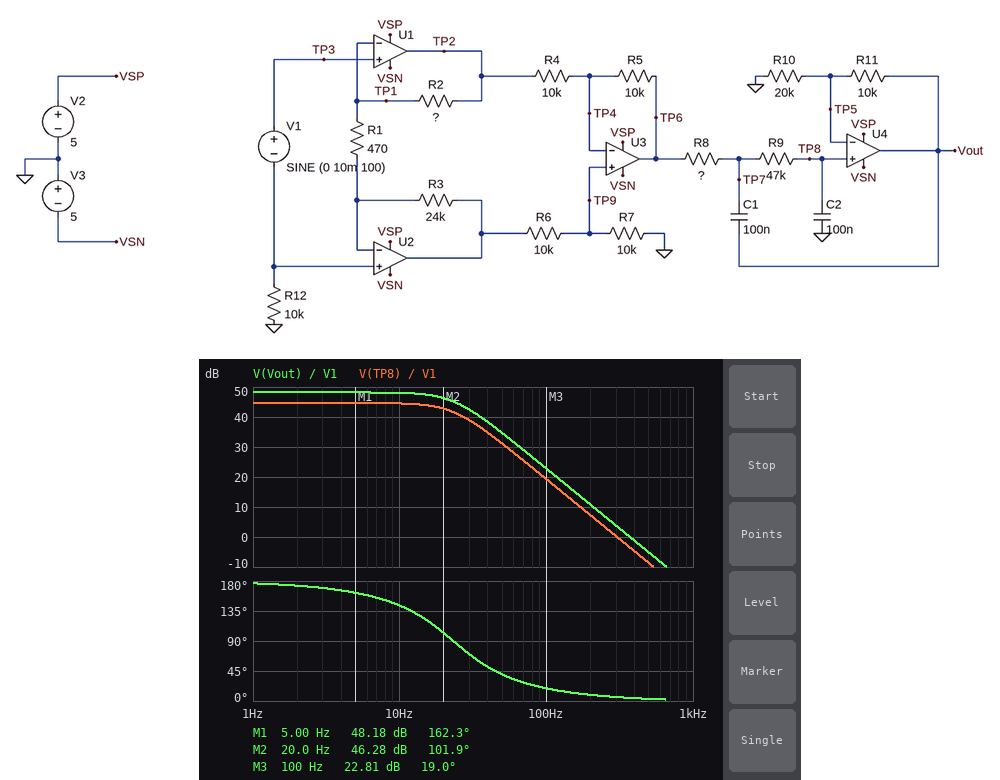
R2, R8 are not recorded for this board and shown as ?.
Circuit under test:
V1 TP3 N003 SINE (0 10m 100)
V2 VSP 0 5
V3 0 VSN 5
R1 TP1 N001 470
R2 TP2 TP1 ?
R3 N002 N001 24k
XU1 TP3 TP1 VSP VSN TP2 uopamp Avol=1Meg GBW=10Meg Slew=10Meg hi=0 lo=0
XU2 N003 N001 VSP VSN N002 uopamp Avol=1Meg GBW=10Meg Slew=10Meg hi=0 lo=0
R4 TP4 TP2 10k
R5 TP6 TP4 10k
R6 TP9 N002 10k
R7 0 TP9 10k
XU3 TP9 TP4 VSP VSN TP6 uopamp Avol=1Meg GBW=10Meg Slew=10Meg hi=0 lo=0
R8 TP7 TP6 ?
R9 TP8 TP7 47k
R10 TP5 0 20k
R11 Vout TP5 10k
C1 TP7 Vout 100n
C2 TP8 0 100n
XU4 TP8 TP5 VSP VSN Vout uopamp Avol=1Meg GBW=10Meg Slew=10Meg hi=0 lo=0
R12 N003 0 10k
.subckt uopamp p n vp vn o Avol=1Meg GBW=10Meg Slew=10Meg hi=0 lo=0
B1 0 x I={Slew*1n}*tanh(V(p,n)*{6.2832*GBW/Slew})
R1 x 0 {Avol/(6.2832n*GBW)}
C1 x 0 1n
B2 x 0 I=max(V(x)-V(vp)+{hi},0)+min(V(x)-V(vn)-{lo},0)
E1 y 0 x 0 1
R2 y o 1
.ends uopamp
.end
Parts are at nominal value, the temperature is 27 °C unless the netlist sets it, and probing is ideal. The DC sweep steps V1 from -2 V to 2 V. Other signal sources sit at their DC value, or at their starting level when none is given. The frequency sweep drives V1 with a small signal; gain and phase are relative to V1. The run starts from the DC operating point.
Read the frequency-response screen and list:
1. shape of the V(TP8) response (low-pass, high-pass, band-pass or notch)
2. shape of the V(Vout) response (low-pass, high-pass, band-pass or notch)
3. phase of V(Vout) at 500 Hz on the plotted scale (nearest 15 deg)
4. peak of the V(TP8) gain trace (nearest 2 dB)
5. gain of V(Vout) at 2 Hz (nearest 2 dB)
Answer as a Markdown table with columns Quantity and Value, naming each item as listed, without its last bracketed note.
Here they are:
| Quantity | Value |
|---|---|
| shape of the V(TP8) response | low-pass |
| shape of the V(Vout) response | low-pass |
| phase of V(Vout) at 500 Hz on the plotted scale | 0 deg |
| peak of the V(TP8) gain trace | 44 dB |
| gain of V(Vout) at 2 Hz | 48 dB |
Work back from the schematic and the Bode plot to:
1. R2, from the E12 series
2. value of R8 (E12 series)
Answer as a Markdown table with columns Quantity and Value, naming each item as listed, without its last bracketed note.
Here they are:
| Quantity | Value |
|---|---|
| R2, from the E12 series | 56 kΩ |
| value of R8 | 100 kΩ |
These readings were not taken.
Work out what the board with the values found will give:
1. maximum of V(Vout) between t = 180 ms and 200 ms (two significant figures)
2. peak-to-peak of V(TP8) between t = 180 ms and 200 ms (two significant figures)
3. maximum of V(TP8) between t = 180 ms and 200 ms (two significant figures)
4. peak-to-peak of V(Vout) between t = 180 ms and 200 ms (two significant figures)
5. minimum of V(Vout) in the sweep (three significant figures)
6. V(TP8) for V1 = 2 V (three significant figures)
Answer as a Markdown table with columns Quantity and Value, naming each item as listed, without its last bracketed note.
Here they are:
| Quantity | Value |
|---|---|
| maximum of V(Vout) between t = 180 ms and 200 ms | 140 mV |
| peak-to-peak of V(TP8) between t = 180 ms and 200 ms | 180 mV |
| maximum of V(TP8) between t = 180 ms and 200 ms | 92 mV |
| peak-to-peak of V(Vout) between t = 180 ms and 200 ms | 280 mV |
| minimum of V(Vout) in the sweep | -5.01 V |
| V(TP8) for V1 = 2 V | -5.01 V |
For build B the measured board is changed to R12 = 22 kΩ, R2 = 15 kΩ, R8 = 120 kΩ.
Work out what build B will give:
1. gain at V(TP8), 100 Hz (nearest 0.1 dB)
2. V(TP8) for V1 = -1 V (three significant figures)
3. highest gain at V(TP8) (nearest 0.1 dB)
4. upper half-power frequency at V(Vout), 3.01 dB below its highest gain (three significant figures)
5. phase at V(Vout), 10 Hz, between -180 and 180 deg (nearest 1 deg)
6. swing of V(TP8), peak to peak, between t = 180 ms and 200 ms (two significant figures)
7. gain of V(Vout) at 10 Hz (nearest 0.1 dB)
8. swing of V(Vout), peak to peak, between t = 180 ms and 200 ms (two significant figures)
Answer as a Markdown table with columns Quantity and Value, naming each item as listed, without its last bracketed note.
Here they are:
| Quantity | Value |
|---|---|
| gain at V(TP8), 100 Hz | 11.5 dB |
| V(TP8) for V1 = -1 V | 5.01 V |
| highest gain at V(TP8) | 38.5 dB |
| upper half-power frequency at V(Vout), 3.01 dB below its highest gain | 21.0 Hz |
| phase at V(Vout), 10 Hz, between -180 and 180 deg | 139 deg |
| swing of V(TP8), peak to peak, between t = 180 ms and 200 ms | 75 mV |
| gain of V(Vout) at 10 Hz | 41.8 dB |
| swing of V(Vout), peak to peak, between t = 180 ms and 200 ms | 110 mV |
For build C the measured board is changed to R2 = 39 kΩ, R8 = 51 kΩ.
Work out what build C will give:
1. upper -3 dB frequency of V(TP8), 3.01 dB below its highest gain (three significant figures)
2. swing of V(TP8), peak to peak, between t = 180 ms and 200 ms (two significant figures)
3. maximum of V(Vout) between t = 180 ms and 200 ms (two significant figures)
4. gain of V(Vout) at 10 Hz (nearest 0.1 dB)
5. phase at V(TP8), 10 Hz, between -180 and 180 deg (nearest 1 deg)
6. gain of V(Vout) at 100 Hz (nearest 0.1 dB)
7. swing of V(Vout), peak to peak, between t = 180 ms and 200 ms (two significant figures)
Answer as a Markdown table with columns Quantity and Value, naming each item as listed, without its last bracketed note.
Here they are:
| Quantity | Value |
|---|---|
| upper -3 dB frequency of V(TP8), 3.01 dB below its highest gain | 31.0 Hz |
| swing of V(TP8), peak to peak, between t = 180 ms and 200 ms | 280 mV |
| maximum of V(Vout) between t = 180 ms and 200 ms | 210 mV |
| gain of V(Vout) at 10 Hz | 46.0 dB |
| phase at V(TP8), 10 Hz, between -180 and 180 deg | 153 deg |
| gain of V(Vout) at 100 Hz | 26.5 dB |
| swing of V(Vout), peak to peak, between t = 180 ms and 200 ms | 420 mV |
